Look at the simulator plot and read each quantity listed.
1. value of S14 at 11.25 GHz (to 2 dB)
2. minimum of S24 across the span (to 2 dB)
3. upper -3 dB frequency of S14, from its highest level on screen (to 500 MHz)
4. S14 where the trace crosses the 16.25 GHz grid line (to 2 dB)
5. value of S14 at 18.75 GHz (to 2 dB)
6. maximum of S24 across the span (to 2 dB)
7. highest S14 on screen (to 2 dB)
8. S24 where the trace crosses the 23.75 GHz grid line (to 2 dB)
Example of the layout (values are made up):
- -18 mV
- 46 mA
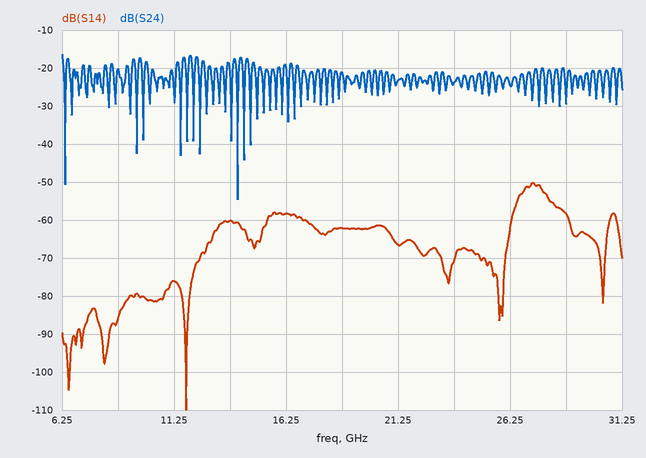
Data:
- -76 dB
- -54 dB
- 28.0 GHz
- -58 dB
- -62 dB
- -16 dB
- -50 dB
- -24 dB
